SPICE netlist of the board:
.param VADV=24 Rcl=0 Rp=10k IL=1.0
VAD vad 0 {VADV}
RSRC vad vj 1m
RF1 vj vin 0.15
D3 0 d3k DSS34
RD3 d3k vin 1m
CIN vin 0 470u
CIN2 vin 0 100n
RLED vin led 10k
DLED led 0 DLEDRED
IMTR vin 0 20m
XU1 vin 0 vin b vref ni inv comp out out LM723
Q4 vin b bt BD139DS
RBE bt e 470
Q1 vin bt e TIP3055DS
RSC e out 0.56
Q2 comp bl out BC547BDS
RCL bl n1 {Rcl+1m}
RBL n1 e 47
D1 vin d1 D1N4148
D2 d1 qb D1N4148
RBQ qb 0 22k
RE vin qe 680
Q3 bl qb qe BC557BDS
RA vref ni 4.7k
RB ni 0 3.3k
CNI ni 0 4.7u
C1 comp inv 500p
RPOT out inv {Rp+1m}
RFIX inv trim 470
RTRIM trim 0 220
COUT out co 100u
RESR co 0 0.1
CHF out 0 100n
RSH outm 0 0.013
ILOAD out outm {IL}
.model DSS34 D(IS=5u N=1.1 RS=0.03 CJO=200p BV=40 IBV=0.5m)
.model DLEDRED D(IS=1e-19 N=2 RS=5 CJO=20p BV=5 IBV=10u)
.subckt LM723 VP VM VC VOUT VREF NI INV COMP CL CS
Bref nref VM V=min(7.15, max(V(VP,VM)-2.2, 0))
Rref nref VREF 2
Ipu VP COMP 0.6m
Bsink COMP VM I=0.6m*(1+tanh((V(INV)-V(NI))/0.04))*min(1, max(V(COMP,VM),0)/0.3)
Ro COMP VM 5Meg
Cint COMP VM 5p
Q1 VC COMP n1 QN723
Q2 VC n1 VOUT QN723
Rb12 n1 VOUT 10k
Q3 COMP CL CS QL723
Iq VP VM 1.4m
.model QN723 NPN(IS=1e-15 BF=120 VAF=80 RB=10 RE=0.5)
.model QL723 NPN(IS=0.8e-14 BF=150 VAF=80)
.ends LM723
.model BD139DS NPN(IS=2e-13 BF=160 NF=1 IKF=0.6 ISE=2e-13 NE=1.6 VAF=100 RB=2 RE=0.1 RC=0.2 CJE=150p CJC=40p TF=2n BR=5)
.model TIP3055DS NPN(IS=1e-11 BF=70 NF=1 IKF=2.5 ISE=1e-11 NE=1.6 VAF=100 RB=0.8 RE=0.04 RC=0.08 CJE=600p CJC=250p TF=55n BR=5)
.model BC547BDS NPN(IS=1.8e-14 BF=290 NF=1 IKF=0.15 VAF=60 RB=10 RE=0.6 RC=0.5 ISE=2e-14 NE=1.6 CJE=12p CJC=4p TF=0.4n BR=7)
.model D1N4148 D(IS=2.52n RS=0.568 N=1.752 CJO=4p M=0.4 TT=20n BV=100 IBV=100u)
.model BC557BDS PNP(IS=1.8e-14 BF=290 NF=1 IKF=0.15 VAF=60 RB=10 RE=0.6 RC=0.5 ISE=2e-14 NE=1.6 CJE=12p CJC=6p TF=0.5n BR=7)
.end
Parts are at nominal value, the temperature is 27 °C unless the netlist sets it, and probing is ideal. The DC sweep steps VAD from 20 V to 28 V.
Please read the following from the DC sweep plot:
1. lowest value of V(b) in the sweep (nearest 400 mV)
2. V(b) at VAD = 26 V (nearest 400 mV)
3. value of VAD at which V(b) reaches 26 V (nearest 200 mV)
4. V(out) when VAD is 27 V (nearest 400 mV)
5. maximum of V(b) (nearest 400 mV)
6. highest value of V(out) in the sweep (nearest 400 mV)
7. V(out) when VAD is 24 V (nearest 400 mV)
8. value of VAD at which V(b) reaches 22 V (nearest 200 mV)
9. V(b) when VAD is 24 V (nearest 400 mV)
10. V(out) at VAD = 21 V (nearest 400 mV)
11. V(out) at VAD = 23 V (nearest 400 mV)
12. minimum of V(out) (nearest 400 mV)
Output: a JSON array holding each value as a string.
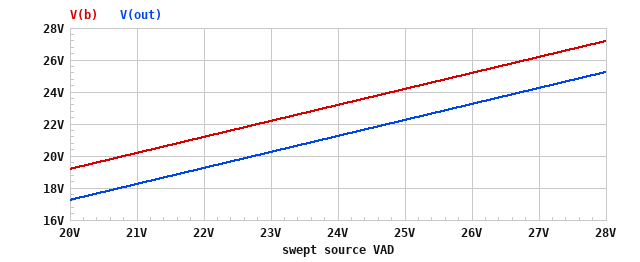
["19.2 V", "25.2 V", "26.8 V", "24.4 V", "27.2 V", "25.2 V", "21.2 V", "22.8 V", "23.2 V", "18.4 V", "20.4 V", "17.2 V"]
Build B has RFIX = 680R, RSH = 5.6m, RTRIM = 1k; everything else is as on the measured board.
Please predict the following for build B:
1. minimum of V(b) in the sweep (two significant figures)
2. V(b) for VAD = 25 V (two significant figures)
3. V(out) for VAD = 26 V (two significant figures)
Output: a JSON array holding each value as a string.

["19 V", "22 V", "20 V"]
